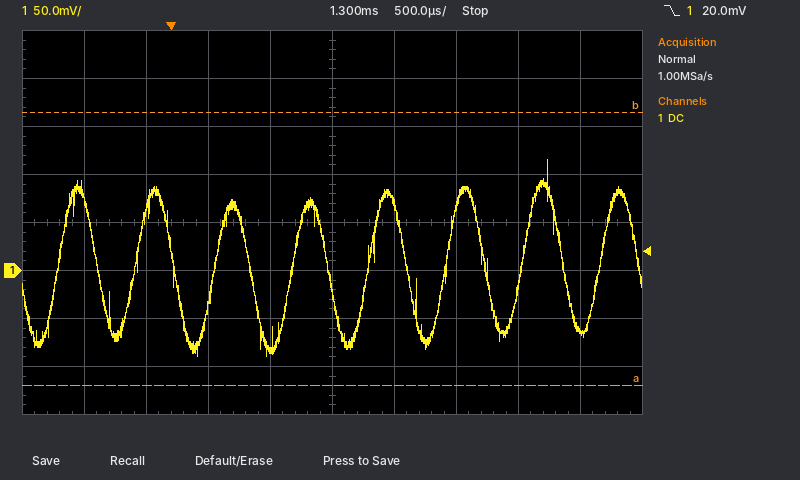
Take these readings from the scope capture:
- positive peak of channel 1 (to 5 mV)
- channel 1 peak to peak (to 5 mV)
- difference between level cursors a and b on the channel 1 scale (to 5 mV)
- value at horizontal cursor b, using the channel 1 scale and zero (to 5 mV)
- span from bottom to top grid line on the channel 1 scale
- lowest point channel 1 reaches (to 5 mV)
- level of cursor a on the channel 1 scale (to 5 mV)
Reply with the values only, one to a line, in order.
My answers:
115 mV
205 mV
285 mV
165 mV
400 mV
-90 mV
-120 mV
